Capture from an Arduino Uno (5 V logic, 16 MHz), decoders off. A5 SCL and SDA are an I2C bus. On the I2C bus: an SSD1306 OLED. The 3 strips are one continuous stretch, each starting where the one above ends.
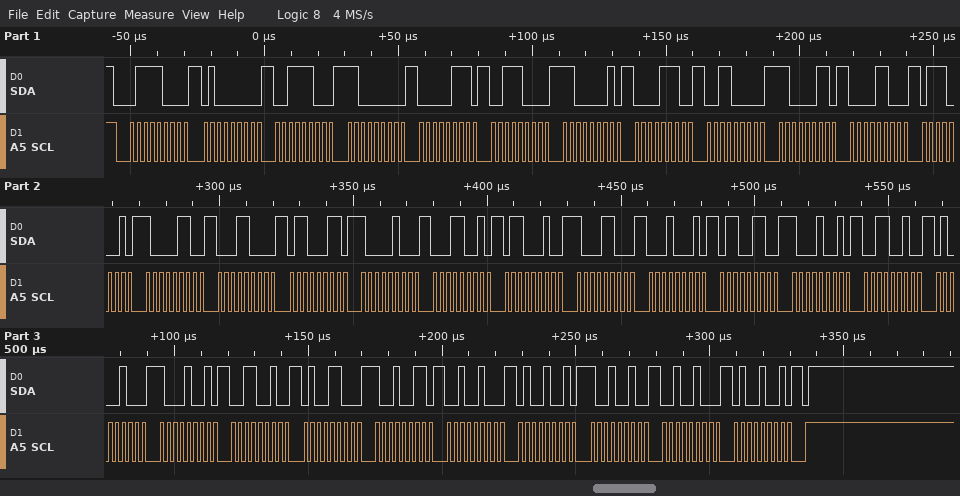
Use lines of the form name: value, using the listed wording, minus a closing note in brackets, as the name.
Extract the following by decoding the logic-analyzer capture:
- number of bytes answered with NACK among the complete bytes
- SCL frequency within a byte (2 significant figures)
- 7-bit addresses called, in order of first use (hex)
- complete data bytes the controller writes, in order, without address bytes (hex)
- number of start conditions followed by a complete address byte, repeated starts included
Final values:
number of bytes answered with NACK among the complete bytes: 0
SCL frequency within a byte: 400 kHz
7-bit addresses called, in order of first use: 0x3C
complete data bytes the controller writes, in order, without address bytes: 40 3C C0 07 38 C1 0E 30 C3 0C 71 86 18 63 84 19 62 8C 11 66 89 32 44 89 32 4C 93 24 49 92 24 49
number of start conditions followed by a complete address byte, repeated starts included: 1
